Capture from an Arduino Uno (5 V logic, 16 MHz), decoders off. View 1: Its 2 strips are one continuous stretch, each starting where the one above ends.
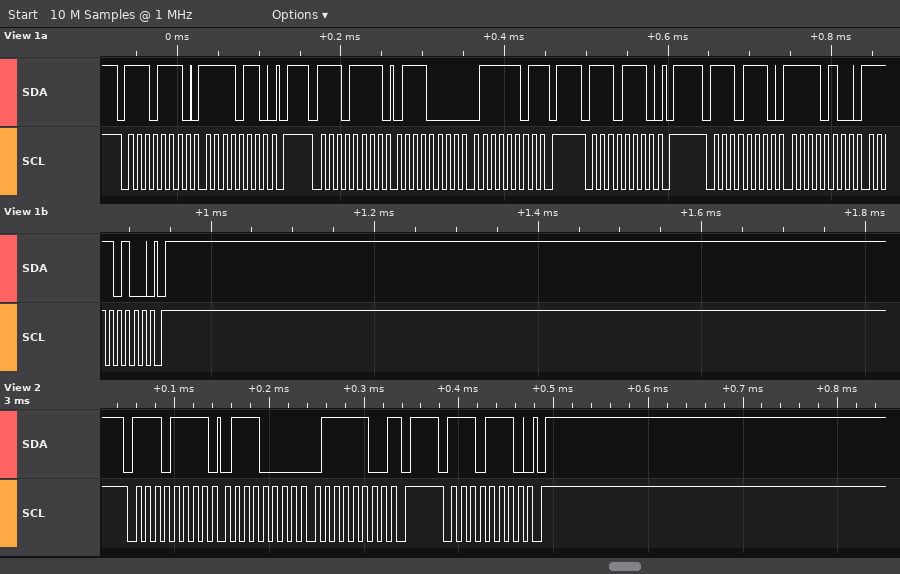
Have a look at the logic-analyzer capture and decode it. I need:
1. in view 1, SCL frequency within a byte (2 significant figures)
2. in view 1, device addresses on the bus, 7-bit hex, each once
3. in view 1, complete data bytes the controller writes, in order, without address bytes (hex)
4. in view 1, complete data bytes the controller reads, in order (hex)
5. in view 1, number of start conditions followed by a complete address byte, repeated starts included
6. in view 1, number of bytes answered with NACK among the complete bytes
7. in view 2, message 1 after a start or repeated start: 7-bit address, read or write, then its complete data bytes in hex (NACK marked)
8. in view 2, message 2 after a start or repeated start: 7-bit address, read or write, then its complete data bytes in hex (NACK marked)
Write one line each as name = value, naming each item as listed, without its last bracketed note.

in view 1, SCL frequency within a byte = 100 kHz
in view 1, device addresses on the bus, 7-bit hex, each once = 0x77
in view 1, complete data bytes the controller writes, in order, without address bytes = F6 F4 F4
in view 1, complete data bytes the controller reads, in order = 70 7D
in view 1, number of start conditions followed by a complete address byte, repeated starts included = 4
in view 1, number of bytes answered with NACK among the complete bytes = 1
in view 2, message 1 after a start or repeated start: 7-bit address, read or write, then its complete data bytes in hex = 0x77 read: 70 7C NACK
in view 2, message 2 after a start or repeated start: 7-bit address, read or write, then its complete data bytes in hex = 0x77 write
